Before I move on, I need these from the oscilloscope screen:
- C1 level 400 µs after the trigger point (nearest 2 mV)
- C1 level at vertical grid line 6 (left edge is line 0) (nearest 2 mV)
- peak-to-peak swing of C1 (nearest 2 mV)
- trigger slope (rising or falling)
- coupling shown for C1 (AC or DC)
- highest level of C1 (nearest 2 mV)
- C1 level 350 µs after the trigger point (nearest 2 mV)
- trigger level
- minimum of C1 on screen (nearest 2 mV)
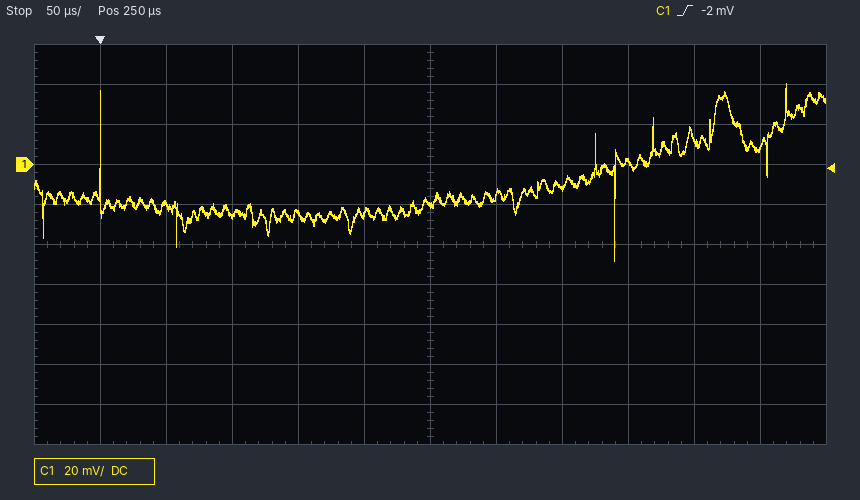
2 mV
-20 mV
88 mV
rising
DC
40 mV
-12 mV
-2 mV
-48 mV
